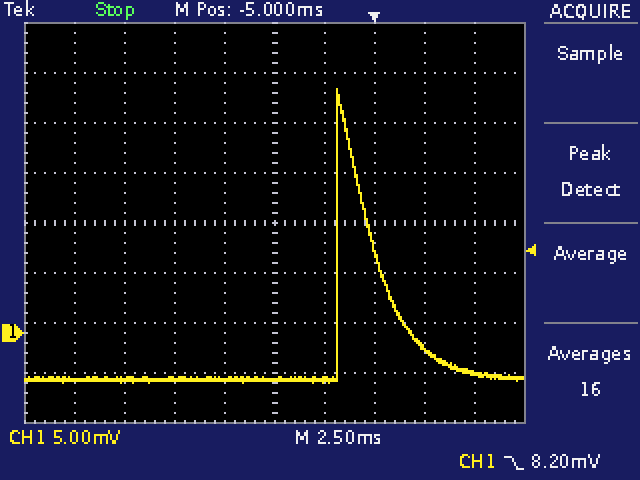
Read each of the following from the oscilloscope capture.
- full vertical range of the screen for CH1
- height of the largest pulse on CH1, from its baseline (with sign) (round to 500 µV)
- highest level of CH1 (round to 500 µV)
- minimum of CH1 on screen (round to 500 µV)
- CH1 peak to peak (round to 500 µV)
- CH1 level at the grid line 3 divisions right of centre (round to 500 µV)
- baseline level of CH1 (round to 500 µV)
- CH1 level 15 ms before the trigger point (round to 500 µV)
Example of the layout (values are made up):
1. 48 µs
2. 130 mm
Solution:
1. 40 mV
2. +29.0 mV
3. 24.5 mV
4. -5.0 mV
5. 29.5 mV
6. -1.5 mV
7. -4.5 mV
8. -4.5 mV
